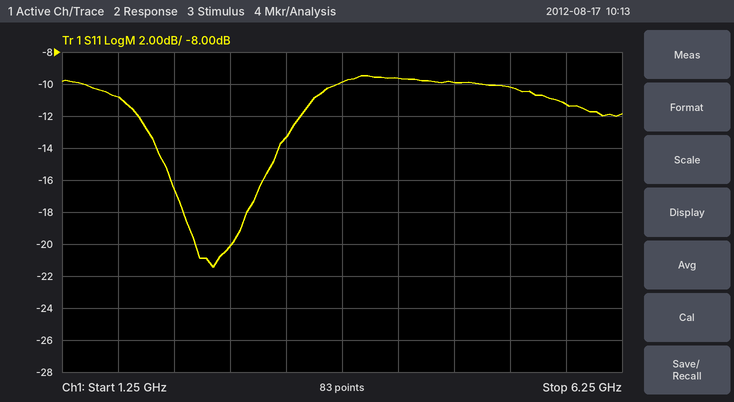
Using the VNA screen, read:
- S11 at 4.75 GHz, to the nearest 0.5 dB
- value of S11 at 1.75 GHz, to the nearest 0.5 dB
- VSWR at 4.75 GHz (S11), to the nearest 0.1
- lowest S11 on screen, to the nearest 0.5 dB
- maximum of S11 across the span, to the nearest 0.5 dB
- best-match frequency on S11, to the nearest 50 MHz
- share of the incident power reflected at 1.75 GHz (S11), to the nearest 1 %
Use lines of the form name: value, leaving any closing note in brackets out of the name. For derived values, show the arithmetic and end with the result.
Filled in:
S11 at 4.75 GHz, to the nearest 0.5 dB: -10.0 dB
value of S11 at 1.75 GHz, to the nearest 0.5 dB: -11.0 dB
VSWR at 4.75 GHz (S11), to the nearest 0.1: |Γ| = 10^(-10/20) = 0.3162; VSWR = (1 + 0.3162)/(1 − 0.3162) ≈ 1.9
lowest S11 on screen, to the nearest 0.5 dB: -21.5 dB
maximum of S11 across the span, to the nearest 0.5 dB: -9.5 dB
best-match frequency on S11, to the nearest 50 MHz: 2.60 GHz
share of the incident power reflected at 1.75 GHz (S11), to the nearest 1 %: 10^(-11/10) ≈ 8 %
